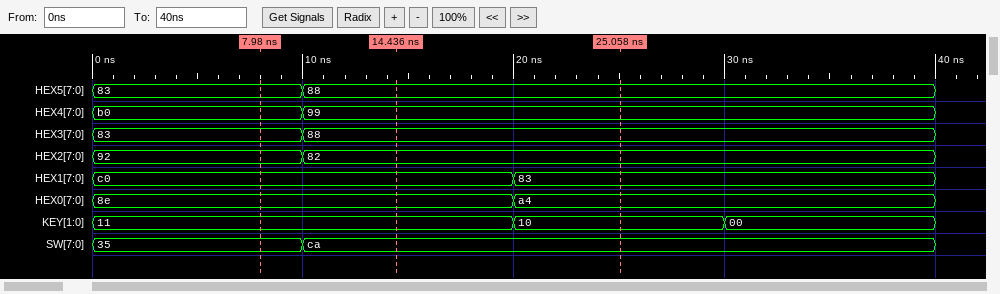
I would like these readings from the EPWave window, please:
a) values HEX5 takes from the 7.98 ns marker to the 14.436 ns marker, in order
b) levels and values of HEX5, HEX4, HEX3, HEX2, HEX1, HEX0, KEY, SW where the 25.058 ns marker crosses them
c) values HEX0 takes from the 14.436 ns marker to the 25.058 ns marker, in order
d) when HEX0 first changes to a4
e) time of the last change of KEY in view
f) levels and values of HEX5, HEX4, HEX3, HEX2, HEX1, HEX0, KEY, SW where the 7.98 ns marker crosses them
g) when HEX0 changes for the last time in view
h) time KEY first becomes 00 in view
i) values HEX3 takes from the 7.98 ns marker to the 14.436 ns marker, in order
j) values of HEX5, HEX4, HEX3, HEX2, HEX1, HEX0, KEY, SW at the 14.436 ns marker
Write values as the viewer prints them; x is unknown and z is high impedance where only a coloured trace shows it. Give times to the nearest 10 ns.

83, 88
HEX5=88, HEX4=99, HEX3=88, HEX2=82, HEX1=83, HEX0=a4, KEY=10, SW=ca
8e, a4
20 ns
30 ns
HEX5=83, HEX4=b0, HEX3=83, HEX2=92, HEX1=c0, HEX0=8e, KEY=11, SW=35
20 ns
30 ns
83, 88
HEX5=88, HEX4=99, HEX3=88, HEX2=82, HEX1=c0, HEX0=8e, KEY=11, SW=ca
